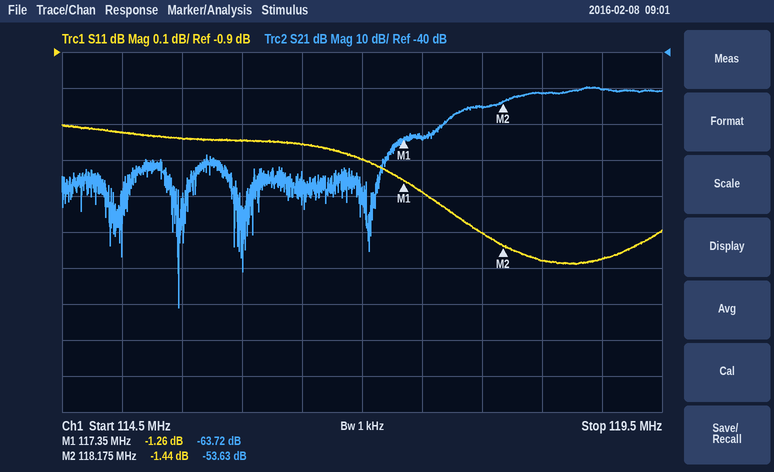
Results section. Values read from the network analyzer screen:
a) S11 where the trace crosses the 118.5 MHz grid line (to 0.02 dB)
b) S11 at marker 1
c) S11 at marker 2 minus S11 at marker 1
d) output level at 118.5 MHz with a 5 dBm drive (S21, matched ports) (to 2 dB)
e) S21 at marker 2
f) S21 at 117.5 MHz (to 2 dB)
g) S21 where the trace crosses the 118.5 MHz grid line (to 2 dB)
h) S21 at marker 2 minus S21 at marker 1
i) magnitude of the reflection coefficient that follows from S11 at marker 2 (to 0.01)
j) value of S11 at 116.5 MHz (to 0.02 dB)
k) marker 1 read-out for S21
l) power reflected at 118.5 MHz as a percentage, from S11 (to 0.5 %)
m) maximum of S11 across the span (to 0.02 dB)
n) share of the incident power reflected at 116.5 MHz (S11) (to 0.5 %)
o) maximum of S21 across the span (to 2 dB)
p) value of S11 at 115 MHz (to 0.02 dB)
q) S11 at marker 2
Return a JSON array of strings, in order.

["-1.48 dB", "-1.26 dB", "-0.18 dB", "-46 dBm", "-53.63 dB", "-64 dB", "-52 dB", "10.09 dB", "0.85", "-1.16 dB", "-63.72 dB", "71.0 %", "-1.10 dB", "76.5 %", "-50 dB", "-1.12 dB", "-1.44 dB"]
